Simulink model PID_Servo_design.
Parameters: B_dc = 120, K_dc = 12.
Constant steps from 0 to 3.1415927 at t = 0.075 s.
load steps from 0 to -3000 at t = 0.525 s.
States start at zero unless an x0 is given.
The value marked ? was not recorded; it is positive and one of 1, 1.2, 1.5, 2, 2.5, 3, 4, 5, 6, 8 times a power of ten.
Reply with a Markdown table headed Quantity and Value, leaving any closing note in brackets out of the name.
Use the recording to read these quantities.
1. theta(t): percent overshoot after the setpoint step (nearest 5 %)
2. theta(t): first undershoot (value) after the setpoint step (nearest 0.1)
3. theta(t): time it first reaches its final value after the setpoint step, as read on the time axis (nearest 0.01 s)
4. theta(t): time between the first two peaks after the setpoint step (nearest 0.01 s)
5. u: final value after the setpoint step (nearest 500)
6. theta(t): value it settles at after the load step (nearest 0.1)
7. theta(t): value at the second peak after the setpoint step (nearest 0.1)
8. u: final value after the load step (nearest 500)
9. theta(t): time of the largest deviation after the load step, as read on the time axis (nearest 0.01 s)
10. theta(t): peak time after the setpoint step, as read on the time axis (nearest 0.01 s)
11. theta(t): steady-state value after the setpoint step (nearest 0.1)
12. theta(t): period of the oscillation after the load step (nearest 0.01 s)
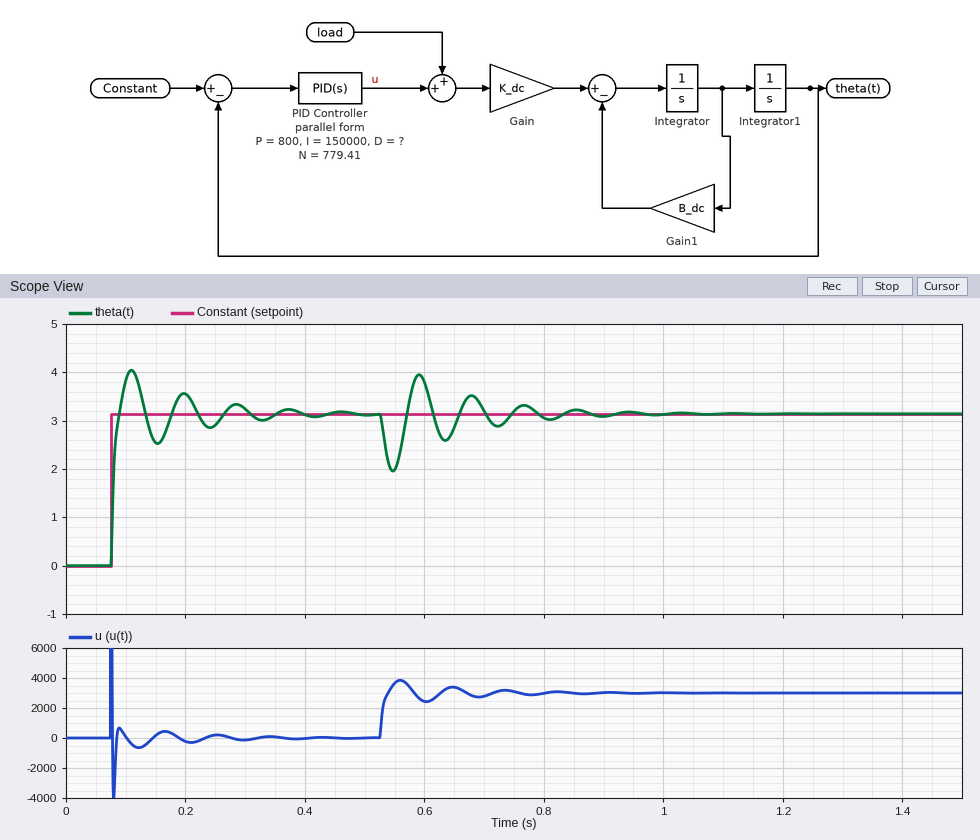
| Quantity | Value |
|---|---|
| theta(t): percent overshoot after the setpoint step | 30 % |
| theta(t): first undershoot (value) after the setpoint step | 2.5 |
| theta(t): time it first reaches its final value after the setpoint step, as read on the time axis | 0.09 s |
| theta(t): time between the first two peaks after the setpoint step | 0.09 s |
| u: final value after the setpoint step | 0 |
| theta(t): value it settles at after the load step | 3.1 |
| theta(t): value at the second peak after the setpoint step | 3.6 |
| u: final value after the load step | 3000 |
| theta(t): time of the largest deviation after the load step, as read on the time axis | 0.55 s |
| theta(t): peak time after the setpoint step, as read on the time axis | 0.11 s |
| theta(t): steady-state value after the setpoint step | 3.1 |
| theta(t): period of the oscillation after the load step | 0.09 s |
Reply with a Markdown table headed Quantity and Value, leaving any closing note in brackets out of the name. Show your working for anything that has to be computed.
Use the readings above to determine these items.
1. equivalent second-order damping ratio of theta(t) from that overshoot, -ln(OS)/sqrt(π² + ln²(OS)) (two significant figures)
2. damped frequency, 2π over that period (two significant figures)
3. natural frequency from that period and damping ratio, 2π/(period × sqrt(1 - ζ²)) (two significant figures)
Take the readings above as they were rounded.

| Quantity | Value |
|---|---|
| equivalent second-order damping ratio of theta(t) from that overshoot, -ln(OS)/sqrt(π² + ln²(OS)) | ln(0.3) = -1.204; 1.204 / sqrt(9.870 + 1.450) = 0.36 |
| damped frequency, 2π over that period | 2π / 0.09 = 70 rad/s |
| natural frequency from that period and damping ratio, 2π/(period × sqrt(1 - ζ²)) | 2π / (0.09 × sqrt(1 - 0.36²)) = 75 rad/s |
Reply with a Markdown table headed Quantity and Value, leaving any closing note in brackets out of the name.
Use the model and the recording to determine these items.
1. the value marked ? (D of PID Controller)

| Quantity | Value |
|---|---|
| the value marked ? | 20 |
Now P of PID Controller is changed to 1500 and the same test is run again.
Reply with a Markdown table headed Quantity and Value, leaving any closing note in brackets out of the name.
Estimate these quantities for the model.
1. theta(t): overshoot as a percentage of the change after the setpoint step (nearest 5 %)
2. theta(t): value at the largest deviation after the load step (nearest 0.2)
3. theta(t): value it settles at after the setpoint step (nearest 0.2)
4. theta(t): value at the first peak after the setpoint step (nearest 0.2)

| Quantity | Value |
|---|---|
| theta(t): overshoot as a percentage of the change after the setpoint step | 20 % |
| theta(t): value at the largest deviation after the load step | 2.2 |
| theta(t): value it settles at after the setpoint step | 3.2 |
| theta(t): value at the first peak after the setpoint step | 3.8 |
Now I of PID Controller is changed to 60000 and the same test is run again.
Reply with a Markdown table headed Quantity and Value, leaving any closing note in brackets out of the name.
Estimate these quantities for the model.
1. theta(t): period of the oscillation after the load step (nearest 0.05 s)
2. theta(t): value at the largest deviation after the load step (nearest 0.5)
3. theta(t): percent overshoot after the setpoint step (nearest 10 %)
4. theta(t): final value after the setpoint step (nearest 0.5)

| Quantity | Value |
|---|---|
| theta(t): period of the oscillation after the load step | 0.15 s |
| theta(t): value at the largest deviation after the load step | 1.5 |
| theta(t): percent overshoot after the setpoint step | 20 % |
| theta(t): final value after the setpoint step | 3.0 |
